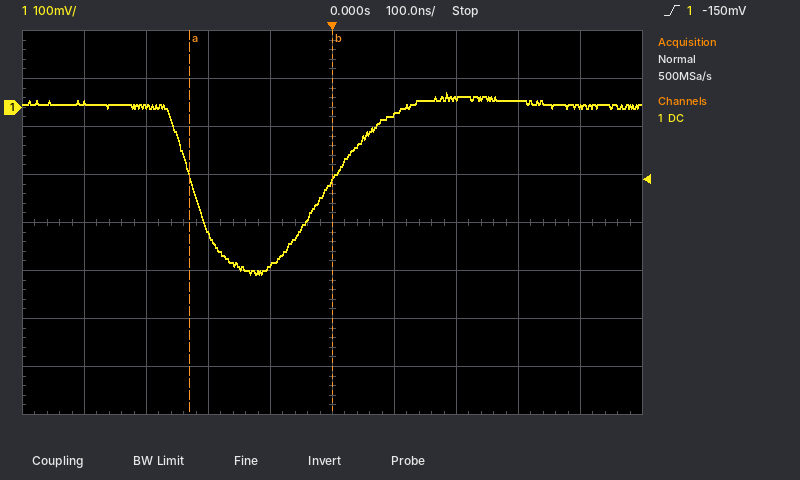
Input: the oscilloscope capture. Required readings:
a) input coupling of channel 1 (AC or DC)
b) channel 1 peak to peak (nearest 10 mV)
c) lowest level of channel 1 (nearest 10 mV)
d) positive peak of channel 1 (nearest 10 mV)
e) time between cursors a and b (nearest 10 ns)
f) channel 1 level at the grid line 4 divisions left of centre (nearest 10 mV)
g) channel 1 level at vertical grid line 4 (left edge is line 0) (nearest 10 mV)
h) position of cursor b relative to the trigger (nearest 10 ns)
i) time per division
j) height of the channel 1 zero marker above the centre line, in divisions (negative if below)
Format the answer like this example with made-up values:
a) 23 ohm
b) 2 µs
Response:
a) DC
b) 380 mV
c) -350 mV
d) 30 mV
e) 230 ns
f) 10 mV
g) -330 mV
h) 0 ns
i) 100 ns
j) +2.4 div
